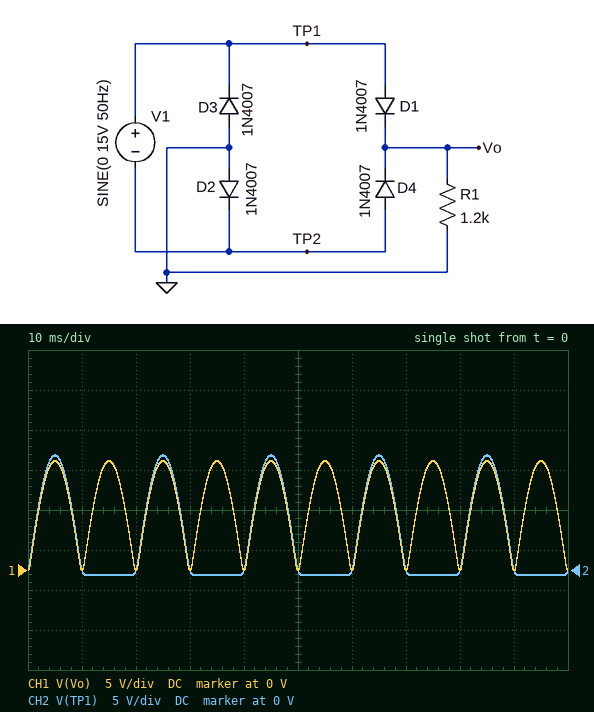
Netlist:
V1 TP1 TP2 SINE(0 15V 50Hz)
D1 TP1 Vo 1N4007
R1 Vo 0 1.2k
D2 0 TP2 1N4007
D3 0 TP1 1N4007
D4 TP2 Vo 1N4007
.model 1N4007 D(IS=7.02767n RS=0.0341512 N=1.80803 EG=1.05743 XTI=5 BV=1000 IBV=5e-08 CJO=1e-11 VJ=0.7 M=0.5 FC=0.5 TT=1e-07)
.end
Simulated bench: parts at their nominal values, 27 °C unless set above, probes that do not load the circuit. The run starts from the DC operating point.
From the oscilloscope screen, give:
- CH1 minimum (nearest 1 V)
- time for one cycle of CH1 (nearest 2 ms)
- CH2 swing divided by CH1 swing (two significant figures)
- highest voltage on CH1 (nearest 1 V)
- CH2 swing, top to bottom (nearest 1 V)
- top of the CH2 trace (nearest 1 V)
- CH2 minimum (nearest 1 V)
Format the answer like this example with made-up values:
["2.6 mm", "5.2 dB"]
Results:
["0 V", "10 ms", "1.1", "14 V", "15 V", "14 V", "-1 V"]
